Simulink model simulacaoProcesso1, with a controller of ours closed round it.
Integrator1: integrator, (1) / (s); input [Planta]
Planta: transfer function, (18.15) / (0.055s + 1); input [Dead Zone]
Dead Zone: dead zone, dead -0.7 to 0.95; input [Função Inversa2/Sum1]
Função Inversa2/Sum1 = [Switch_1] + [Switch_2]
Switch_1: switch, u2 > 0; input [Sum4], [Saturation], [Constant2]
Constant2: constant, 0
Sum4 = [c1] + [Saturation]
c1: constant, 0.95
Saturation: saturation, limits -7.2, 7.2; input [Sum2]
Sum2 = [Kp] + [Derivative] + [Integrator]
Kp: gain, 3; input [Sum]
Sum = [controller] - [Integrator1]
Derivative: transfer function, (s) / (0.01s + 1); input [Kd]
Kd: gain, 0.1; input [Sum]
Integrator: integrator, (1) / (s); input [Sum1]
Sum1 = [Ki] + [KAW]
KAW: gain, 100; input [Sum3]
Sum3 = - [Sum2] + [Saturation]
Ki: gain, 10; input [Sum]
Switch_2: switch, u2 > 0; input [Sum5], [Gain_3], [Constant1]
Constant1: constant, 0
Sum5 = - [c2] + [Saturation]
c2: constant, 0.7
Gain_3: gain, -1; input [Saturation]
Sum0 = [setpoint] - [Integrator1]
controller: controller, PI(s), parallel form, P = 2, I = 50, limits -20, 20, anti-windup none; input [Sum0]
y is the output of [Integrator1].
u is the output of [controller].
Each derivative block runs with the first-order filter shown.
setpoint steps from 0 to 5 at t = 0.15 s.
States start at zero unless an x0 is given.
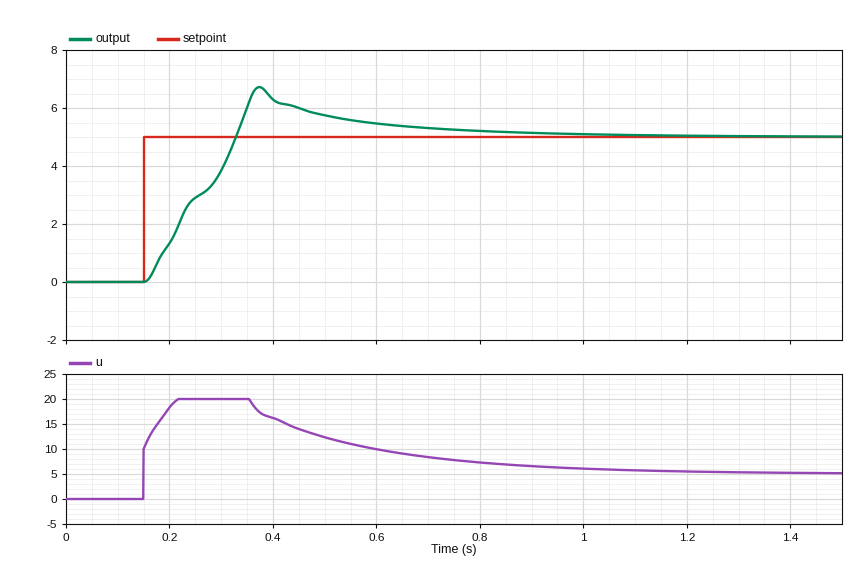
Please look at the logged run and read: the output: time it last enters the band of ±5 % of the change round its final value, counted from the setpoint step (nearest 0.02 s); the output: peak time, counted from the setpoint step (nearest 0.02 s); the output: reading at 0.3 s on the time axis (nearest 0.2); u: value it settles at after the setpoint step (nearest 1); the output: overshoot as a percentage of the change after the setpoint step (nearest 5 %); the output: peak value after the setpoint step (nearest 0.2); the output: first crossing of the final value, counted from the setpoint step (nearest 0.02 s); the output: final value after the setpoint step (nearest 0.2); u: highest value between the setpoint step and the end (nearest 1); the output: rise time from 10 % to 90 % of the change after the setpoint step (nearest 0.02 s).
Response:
0.60 s
0.22 s
3.8
5
35 %
6.8
0.18 s
5.0
20
0.14 s
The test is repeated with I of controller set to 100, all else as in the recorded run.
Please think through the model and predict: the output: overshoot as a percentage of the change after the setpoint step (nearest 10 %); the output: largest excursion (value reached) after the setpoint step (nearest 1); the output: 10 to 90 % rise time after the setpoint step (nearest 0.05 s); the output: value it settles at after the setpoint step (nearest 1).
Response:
140 %
12
0.20 s
5
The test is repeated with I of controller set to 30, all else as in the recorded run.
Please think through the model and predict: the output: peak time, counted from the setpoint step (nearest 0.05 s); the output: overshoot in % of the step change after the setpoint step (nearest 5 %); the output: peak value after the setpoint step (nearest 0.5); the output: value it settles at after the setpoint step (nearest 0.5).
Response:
0.35 s
15 %
6.0
5.0
